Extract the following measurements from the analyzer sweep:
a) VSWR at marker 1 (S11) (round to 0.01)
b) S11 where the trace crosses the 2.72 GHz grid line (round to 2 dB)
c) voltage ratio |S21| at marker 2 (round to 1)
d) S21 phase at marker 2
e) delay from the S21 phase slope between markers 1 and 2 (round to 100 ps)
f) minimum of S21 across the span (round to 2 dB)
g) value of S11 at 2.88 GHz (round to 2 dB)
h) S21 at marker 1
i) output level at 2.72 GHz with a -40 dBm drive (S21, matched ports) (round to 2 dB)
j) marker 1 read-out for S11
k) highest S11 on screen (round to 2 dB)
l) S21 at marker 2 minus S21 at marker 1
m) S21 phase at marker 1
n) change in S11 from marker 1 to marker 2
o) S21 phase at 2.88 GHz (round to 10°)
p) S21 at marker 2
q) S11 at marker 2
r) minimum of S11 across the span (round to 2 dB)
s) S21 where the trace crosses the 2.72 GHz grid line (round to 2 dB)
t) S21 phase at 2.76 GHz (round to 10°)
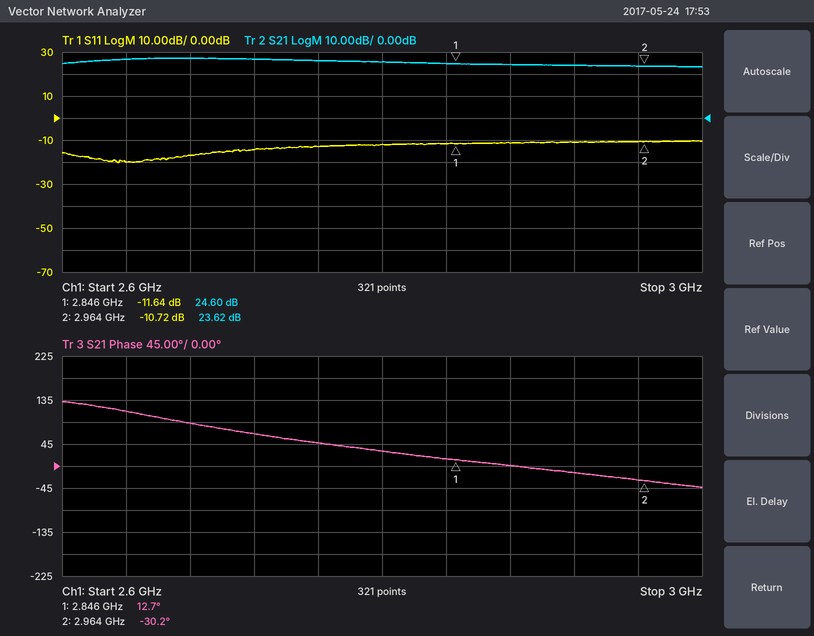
1.71
-14 dB
15
-30.2°
1.0 ns
24 dB
-12 dB
24.60 dB
-14 dBm
-11.64 dB
-10 dB
-0.98 dB
12.7°
0.92 dB
0°
23.62 dB
-10.72 dB
-20 dB
26 dB
50°
